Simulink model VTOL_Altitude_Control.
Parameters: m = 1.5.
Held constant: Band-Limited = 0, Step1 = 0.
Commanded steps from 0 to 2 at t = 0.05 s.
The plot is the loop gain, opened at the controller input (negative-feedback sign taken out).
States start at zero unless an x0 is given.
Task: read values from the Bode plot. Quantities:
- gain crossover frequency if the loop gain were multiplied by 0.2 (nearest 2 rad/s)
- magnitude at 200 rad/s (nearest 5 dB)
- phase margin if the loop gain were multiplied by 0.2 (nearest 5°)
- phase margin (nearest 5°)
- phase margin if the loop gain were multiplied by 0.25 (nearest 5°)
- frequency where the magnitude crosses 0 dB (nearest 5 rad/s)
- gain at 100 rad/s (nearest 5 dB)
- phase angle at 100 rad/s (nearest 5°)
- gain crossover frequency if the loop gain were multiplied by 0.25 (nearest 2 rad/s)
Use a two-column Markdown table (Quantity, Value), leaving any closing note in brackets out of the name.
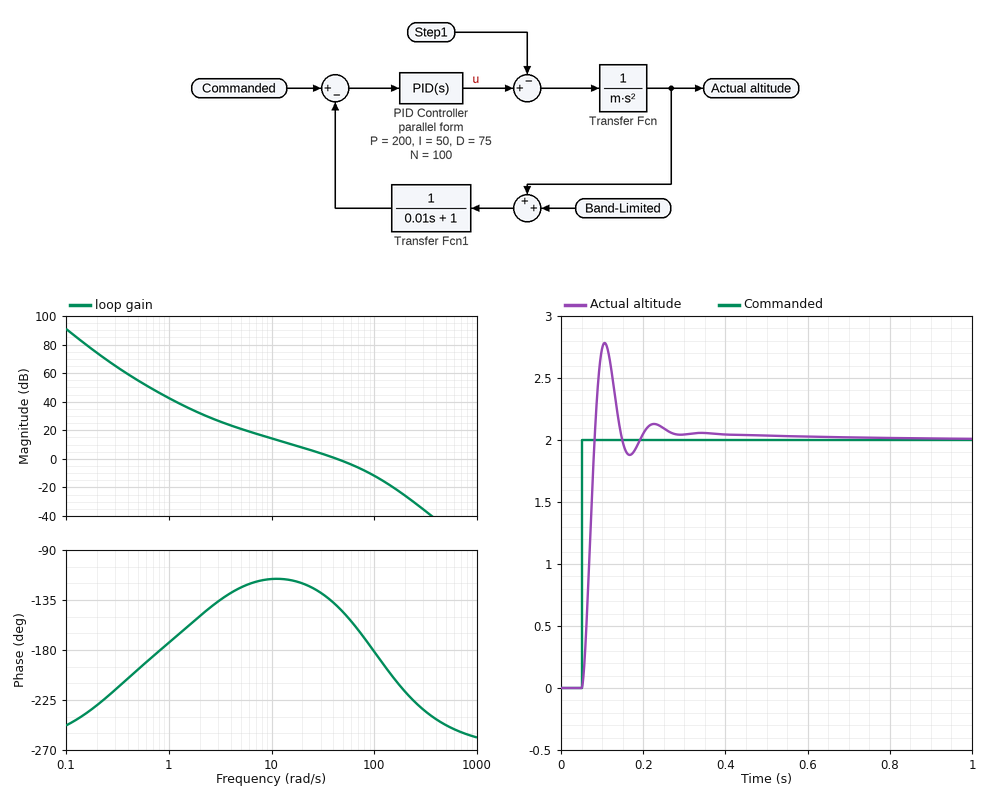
| Quantity | Value |
|---|---|
| gain crossover frequency if the loop gain were multiplied by 0.2 | 10 rad/s |
| magnitude at 200 rad/s | -25 dB |
| phase margin if the loop gain were multiplied by 0.2 | 65° |
| phase margin | 40° |
| phase margin if the loop gain were multiplied by 0.25 | 65° |
| frequency where the magnitude crosses 0 dB | 45 rad/s |
| gain at 100 rad/s | -10 dB |
| phase angle at 100 rad/s | -180° |
| gain crossover frequency if the loop gain were multiplied by 0.25 | 12 rad/s |
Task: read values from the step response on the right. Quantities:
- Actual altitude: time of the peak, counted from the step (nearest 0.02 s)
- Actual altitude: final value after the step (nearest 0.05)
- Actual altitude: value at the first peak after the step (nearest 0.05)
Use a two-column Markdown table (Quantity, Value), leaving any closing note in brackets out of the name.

| Quantity | Value |
|---|---|
| Actual altitude: time of the peak, counted from the step | 0.06 s |
| Actual altitude: final value after the step | 2.00 |
| Actual altitude: value at the first peak after the step | 2.80 |
